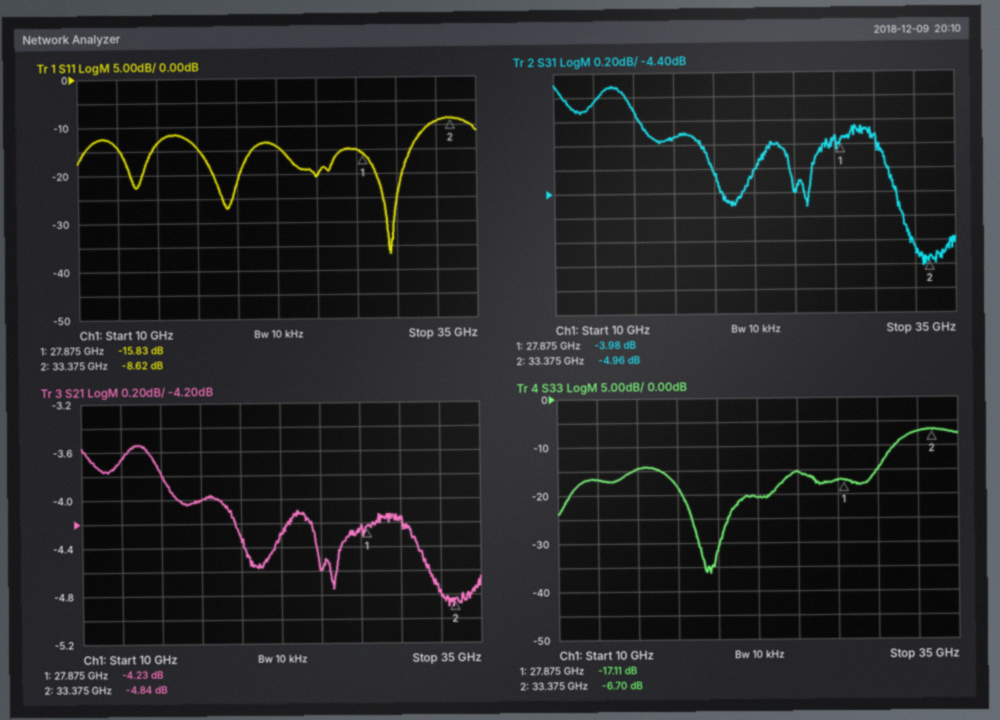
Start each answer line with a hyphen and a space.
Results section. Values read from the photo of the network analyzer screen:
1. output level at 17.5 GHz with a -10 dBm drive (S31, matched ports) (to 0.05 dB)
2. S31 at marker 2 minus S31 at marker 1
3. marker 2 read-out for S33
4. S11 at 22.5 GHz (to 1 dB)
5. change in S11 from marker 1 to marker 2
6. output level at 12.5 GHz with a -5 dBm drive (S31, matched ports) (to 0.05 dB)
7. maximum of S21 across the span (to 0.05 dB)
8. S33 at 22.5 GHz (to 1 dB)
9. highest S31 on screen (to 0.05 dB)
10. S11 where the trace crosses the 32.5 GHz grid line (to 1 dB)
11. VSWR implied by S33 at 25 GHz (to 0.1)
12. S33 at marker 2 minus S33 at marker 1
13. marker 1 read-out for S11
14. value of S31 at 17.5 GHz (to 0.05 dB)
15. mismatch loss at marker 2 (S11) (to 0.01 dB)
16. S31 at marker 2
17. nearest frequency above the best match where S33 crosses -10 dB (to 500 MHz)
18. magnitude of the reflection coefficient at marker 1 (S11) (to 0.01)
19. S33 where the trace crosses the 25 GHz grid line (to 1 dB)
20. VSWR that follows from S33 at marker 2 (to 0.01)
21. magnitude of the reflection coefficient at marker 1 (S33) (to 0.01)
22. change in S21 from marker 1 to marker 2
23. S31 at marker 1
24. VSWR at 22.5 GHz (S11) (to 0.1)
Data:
- -13.95 dBm
- -0.98 dB
- -6.70 dB
- -14 dB
- 7.21 dB
- -8.65 dBm
- -3.55 dB
- -21 dB
- -3.50 dB
- -9 dB
- 1.4
- 10.41 dB
- -15.83 dB
- -3.95 dB
- 0.64 dB
- -4.96 dB
- 31.0 GHz
- 0.16
- -15 dB
- 2.72
- 0.14
- -0.61 dB
- -3.98 dB
- 1.5
